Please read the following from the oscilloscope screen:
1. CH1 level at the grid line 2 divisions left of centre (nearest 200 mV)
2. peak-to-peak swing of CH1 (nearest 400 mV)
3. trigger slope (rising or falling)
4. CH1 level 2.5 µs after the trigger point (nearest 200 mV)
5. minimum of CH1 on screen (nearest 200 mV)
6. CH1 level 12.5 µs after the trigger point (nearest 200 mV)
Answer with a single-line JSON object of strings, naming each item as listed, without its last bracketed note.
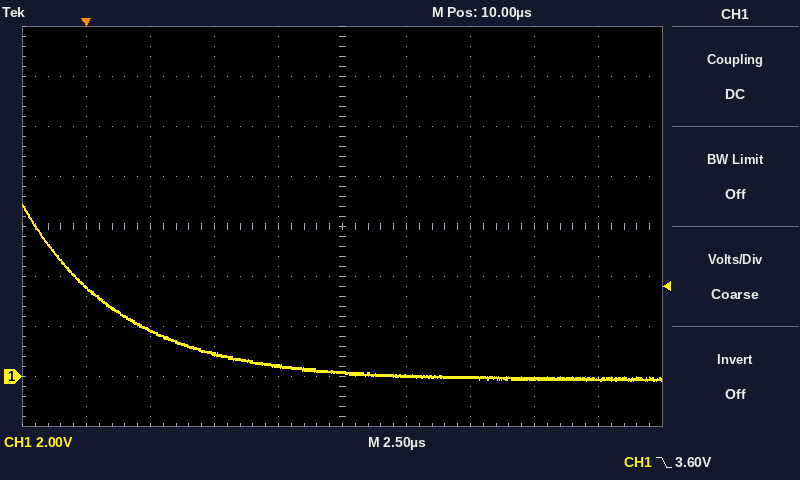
{"CH1 level at the grid line 2 divisions left of centre": "1.0 V", "peak-to-peak swing of CH1": "7.2 V", "trigger slope": "falling", "CH1 level 2.5 µs after the trigger point": "1.8 V", "minimum of CH1 on screen": "-200 mV", "CH1 level 12.5 µs after the trigger point": "0.0 V"}
